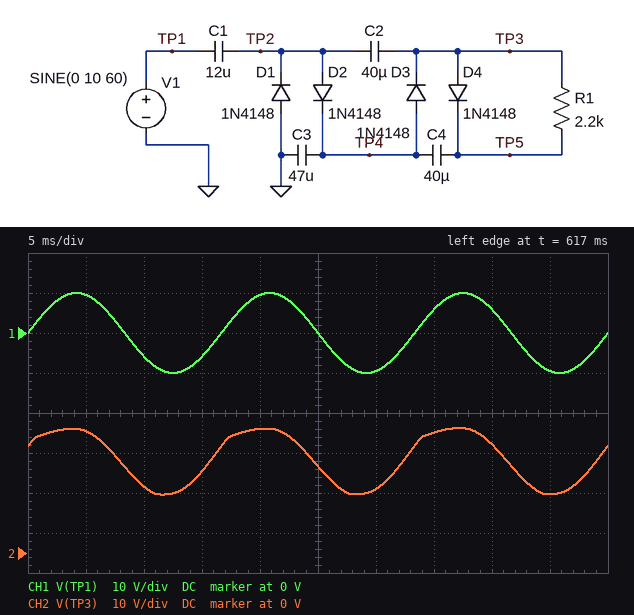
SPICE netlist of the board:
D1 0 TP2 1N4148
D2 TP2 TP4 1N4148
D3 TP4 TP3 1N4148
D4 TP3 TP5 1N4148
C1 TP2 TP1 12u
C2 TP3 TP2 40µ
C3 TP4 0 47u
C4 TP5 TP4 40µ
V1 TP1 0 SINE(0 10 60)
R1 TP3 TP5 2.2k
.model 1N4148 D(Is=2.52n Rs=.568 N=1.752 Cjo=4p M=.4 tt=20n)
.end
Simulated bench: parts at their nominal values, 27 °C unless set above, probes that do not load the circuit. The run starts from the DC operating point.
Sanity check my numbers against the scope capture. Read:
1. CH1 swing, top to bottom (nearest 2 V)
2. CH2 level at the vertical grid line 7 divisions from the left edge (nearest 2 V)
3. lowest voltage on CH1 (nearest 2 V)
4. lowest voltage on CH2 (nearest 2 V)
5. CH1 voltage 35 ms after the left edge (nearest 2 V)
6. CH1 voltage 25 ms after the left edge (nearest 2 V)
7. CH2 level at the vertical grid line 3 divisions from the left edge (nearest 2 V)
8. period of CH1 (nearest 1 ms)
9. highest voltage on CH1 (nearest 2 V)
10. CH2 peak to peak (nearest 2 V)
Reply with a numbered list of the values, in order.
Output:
1. 20 V
2. 30 V
3. -10 V
4. 14 V
5. 6 V
6. 0 V
7. 20 V
8. 17 ms
9. 10 V
10. 16 V
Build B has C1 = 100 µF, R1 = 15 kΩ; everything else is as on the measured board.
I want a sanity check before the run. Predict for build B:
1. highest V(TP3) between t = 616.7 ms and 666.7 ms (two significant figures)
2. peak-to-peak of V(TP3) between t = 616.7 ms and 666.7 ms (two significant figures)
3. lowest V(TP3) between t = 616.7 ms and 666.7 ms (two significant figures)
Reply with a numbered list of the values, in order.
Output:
1. 38 V
2. 20 V
3. 18 V
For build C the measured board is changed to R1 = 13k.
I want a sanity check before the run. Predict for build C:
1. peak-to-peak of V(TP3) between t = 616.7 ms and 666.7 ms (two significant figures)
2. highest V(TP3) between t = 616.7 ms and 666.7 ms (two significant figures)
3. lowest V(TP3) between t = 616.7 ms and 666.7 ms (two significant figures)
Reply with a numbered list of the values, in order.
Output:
1. 19 V
2. 35 V
3. 17 V
